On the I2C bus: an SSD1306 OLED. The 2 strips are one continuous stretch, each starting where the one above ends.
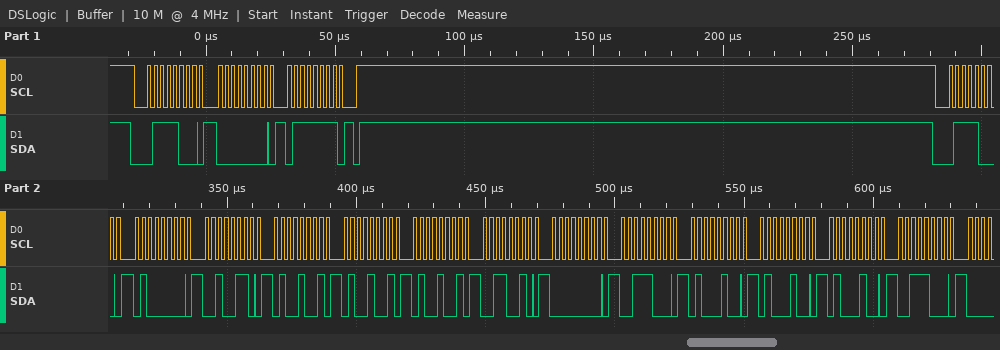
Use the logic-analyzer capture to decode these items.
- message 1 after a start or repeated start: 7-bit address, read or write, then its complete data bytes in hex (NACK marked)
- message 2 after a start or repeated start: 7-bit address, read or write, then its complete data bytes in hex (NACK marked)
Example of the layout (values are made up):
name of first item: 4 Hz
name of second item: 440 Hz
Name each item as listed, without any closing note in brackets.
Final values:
message 1 after a start or repeated start: 7-bit address, read or write, then its complete data bytes in hex: 0x3C write: 00 7F
message 2 after a start or repeated start: 7-bit address, read or write, then its complete data bytes in hex: 0x3C write: 40 26 49 49 49 32 00 38 44 44 44 38
